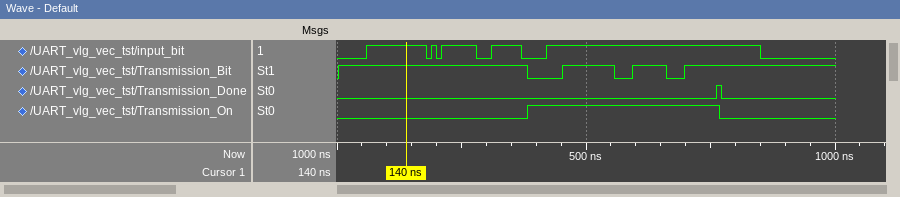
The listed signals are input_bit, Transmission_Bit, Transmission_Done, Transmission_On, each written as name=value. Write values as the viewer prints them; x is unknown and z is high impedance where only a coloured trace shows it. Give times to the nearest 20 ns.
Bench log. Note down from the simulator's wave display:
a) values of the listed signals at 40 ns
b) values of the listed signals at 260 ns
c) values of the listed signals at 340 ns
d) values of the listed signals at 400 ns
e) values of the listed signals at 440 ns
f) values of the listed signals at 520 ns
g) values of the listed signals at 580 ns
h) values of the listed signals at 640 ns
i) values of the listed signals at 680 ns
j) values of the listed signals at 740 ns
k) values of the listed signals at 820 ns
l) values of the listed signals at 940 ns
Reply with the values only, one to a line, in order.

input_bit=0, Transmission_Bit=1, Transmission_Done=0, Transmission_On=0
input_bit=1, Transmission_Bit=1, Transmission_Done=0, Transmission_On=0
input_bit=1, Transmission_Bit=1, Transmission_Done=0, Transmission_On=0
input_bit=0, Transmission_Bit=0, Transmission_Done=0, Transmission_On=1
input_bit=1, Transmission_Bit=0, Transmission_Done=0, Transmission_On=1
input_bit=1, Transmission_Bit=1, Transmission_Done=0, Transmission_On=1
input_bit=1, Transmission_Bit=0, Transmission_Done=0, Transmission_On=1
input_bit=1, Transmission_Bit=1, Transmission_Done=0, Transmission_On=1
input_bit=1, Transmission_Bit=0, Transmission_Done=0, Transmission_On=1
input_bit=1, Transmission_Bit=1, Transmission_Done=0, Transmission_On=1
input_bit=1, Transmission_Bit=1, Transmission_Done=0, Transmission_On=0
input_bit=0, Transmission_Bit=1, Transmission_Done=0, Transmission_On=0
